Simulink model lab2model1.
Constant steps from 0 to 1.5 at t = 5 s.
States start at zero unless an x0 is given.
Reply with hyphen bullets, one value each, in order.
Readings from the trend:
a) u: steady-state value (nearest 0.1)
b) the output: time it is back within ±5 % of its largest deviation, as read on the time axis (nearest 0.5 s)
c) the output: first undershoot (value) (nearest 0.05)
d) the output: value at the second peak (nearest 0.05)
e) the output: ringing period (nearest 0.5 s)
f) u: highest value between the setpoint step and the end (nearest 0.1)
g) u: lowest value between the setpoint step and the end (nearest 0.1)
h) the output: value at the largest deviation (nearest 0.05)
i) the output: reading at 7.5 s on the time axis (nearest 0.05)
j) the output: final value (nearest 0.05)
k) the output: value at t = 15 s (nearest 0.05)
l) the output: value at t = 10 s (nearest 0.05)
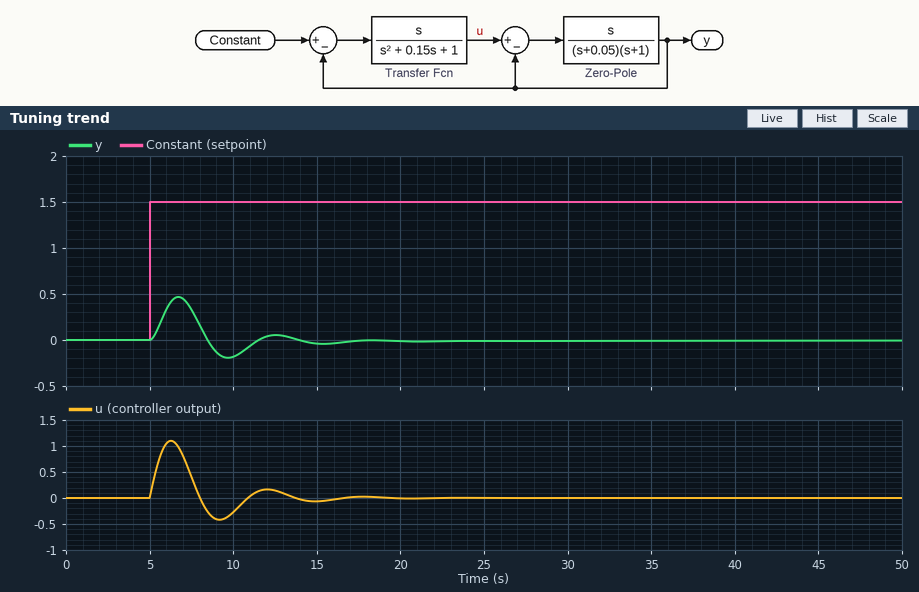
- 0.0
- 16.5 s
- -0.20
- 0.05
- 6.0 s
- 1.1
- -0.4
- 0.45
- 0.35
- 0.00
- -0.05
- -0.20
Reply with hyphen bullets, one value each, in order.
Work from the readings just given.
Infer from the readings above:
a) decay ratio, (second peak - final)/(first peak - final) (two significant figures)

- 0.11
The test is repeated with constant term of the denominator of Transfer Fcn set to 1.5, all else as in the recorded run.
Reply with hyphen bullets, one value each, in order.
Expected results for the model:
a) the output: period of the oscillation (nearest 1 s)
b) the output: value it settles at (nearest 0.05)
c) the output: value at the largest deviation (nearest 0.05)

- 5 s
- 0.00
- 0.40
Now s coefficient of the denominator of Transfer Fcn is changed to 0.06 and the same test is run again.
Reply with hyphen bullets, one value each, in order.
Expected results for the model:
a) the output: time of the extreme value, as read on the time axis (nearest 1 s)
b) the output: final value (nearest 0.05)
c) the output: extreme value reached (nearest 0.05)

- 7 s
- 0.00
- 0.50
